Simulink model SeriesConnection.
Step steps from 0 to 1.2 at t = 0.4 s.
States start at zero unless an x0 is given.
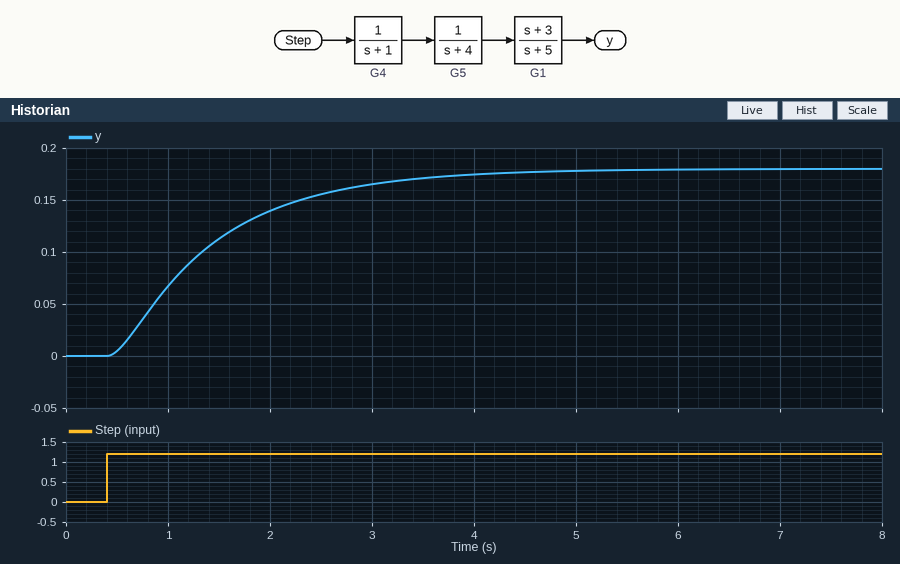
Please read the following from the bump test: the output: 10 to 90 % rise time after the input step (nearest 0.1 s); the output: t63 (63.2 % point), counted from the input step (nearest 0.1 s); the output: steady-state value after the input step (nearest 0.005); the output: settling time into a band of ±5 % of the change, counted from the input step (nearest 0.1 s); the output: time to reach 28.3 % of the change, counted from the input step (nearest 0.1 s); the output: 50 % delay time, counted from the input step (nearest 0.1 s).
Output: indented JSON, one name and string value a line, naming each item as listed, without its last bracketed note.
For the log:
{
  "the output: 10 to 90 % rise time after the input step": "2.2 s",
  "the output: t63 (63.2 % point), counted from the input step": "1.1 s",
  "the output: steady-state value after the input step": "0.180",
  "the output: settling time into a band of ±5 % of the change, counted from the input step": "3.1 s",
  "the output: time to reach 28.3 % of the change, counted from the input step": "0.5 s",
  "the output: 50 % delay time, counted from the input step": "0.8 s"
}
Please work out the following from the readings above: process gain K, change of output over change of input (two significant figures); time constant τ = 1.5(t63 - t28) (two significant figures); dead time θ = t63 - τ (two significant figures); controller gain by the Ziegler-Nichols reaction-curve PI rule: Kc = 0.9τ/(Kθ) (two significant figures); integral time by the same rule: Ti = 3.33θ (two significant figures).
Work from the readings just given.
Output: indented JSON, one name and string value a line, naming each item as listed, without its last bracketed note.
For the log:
{
  "process gain K, change of output over change of input": "0.15",
  "time constant τ = 1.5(t63 - t28)": "0.90 s",
  "dead time θ = t63 - τ": "0.20 s",
  "controller gain by the Ziegler-Nichols reaction-curve PI rule: Kc = 0.9τ/(Kθ)": "27",
  "integral time by the same rule: Ti = 3.33θ": "0.67 s"
}
